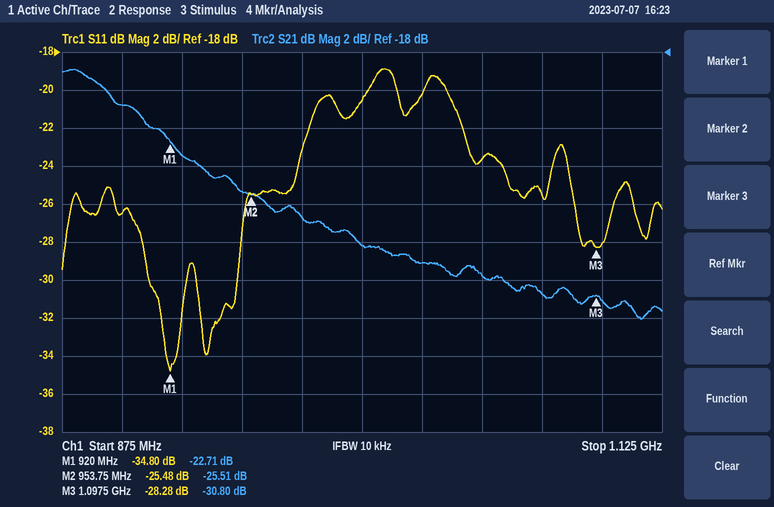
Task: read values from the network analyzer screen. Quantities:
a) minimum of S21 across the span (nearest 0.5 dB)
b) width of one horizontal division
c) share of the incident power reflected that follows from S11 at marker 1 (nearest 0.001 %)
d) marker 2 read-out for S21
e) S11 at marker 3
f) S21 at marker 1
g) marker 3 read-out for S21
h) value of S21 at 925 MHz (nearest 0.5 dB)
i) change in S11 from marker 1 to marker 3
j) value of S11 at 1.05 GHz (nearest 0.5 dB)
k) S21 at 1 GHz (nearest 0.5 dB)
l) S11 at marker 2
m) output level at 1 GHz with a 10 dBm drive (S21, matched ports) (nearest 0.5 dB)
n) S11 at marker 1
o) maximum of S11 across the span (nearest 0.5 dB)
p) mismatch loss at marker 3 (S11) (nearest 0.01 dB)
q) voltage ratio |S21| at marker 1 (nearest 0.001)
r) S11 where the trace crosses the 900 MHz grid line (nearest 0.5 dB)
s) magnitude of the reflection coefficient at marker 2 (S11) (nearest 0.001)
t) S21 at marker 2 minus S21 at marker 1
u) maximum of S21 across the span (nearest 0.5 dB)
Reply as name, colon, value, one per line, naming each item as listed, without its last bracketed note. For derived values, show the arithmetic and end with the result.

minimum of S21 across the span: -32.0 dB
width of one horizontal division: 25 MHz
share of the incident power reflected that follows from S11 at marker 1: 10^(-34.8/10) ≈ 0.033 %
marker 2 read-out for S21: -25.51 dB
S11 at marker 3: -28.28 dB
S21 at marker 1: -22.71 dB
marker 3 read-out for S21: -30.80 dB
value of S21 at 925 MHz: -23.5 dB
change in S11 from marker 1 to marker 3: -28.28 − (-34.8) = 6.52 dB
value of S11 at 1.05 GHz: -23.5 dB
S21 at 1 GHz: -28.0 dB
S11 at marker 2: -25.48 dB
output level at 1 GHz with a 10 dBm drive (S21, matched ports): 10 dBm + (-28.0 dB) = -18.0 dBm
S11 at marker 1: -34.80 dB
maximum of S11 across the span: -19.0 dB
mismatch loss at marker 3 (S11): −10 log10(1 − 10^(-28.28/10)) ≈ 0.01 dB
voltage ratio |S21| at marker 1: 10^(-22.71/20) ≈ 0.073
S11 where the trace crosses the 900 MHz grid line: -26.5 dB
magnitude of the reflection coefficient at marker 2 (S11): 10^(-25.48/20) ≈ 0.053
S21 at marker 2 minus S21 at marker 1: -25.51 − (-22.71) = -2.80 dB
maximum of S21 across the span: -19.0 dB
